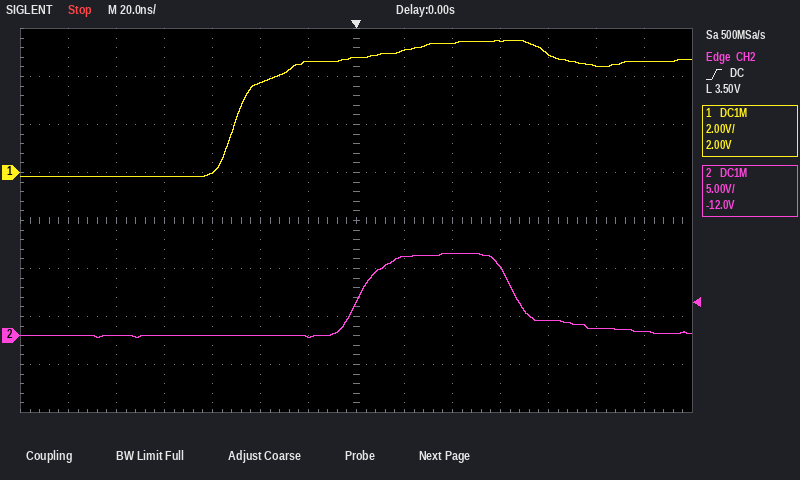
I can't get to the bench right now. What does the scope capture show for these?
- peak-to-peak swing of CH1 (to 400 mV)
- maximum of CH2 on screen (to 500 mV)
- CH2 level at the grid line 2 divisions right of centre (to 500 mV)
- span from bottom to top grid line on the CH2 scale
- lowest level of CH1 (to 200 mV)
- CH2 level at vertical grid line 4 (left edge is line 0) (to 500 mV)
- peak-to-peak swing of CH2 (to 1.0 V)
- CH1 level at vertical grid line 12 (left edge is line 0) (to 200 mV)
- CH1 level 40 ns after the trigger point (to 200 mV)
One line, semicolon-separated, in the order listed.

5.6 V; 8.5 V; 8.5 V; 40 V; -200 mV; 0.0 V; 9.0 V; 4.4 V; 5.4 V
